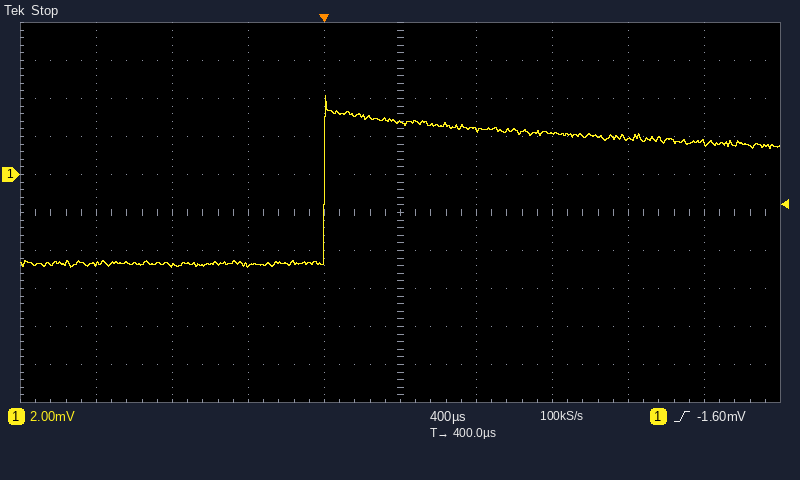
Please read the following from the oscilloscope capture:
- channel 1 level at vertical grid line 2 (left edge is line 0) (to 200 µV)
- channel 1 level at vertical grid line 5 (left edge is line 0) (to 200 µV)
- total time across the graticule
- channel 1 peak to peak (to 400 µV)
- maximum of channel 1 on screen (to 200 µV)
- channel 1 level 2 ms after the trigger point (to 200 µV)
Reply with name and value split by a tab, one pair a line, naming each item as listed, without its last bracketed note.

channel 1 level at vertical grid line 2 (left edge is line 0)	-4.8 mV
channel 1 level at vertical grid line 5 (left edge is line 0)	2.8 mV
total time across the graticule	4 ms
channel 1 peak to peak	9.2 mV
maximum of channel 1 on screen	4.2 mV
channel 1 level 2 ms after the trigger point	1.6 mV
